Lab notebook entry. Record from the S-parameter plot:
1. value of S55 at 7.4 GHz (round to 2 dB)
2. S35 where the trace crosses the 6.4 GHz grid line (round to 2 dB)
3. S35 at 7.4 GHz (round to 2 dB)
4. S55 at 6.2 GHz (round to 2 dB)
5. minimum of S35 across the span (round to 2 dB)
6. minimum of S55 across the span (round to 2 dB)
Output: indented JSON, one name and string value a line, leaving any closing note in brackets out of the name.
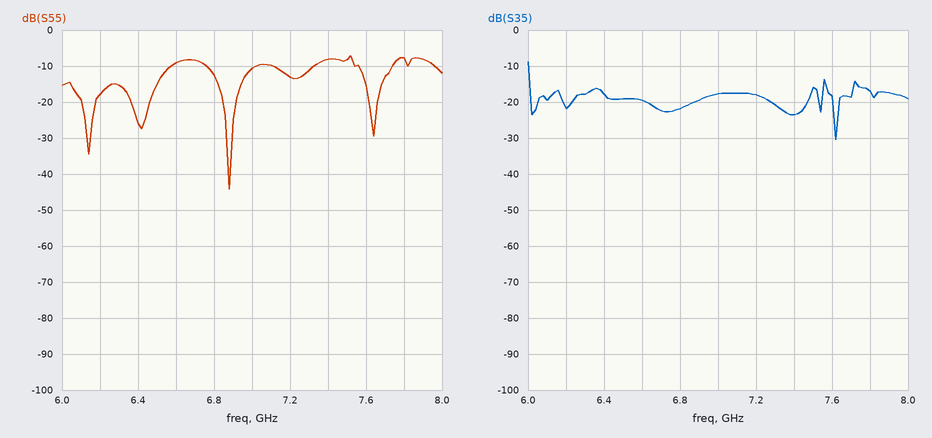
{
  "value of S55 at 7.4 GHz": "-8 dB",
  "S35 where the trace crosses the 6.4 GHz grid line": "-18 dB",
  "S35 at 7.4 GHz": "-24 dB",
  "S55 at 6.2 GHz": "-18 dB",
  "minimum of S35 across the span": "-30 dB",
  "minimum of S55 across the span": "-44 dB"
}
